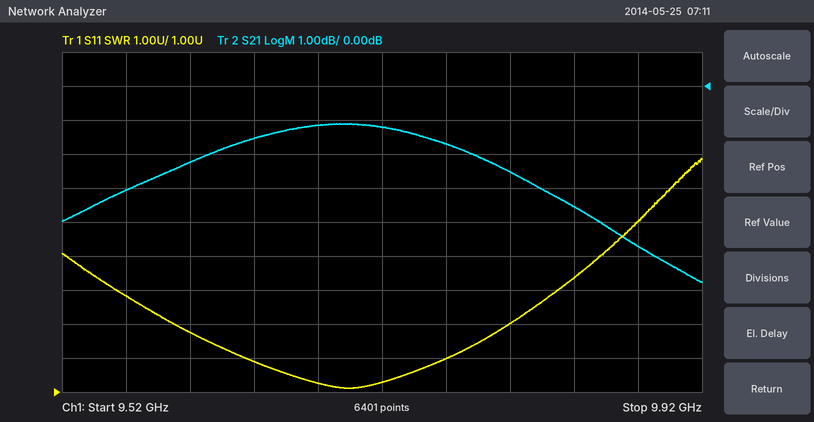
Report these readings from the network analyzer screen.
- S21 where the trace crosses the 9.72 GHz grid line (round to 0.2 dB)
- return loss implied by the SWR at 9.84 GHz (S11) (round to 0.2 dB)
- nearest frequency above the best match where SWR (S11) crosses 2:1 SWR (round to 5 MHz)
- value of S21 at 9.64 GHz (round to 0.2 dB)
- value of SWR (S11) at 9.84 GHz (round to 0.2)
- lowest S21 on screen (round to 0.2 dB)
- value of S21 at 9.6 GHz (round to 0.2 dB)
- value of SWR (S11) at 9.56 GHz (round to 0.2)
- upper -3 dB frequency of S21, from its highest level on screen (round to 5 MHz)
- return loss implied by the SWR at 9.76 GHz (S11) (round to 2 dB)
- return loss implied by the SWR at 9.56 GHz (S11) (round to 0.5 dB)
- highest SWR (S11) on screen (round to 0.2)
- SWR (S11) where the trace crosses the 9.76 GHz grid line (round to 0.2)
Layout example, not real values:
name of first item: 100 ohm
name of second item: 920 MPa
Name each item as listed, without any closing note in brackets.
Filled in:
S21 where the trace crosses the 9.72 GHz grid line: -1.2 dB
return loss implied by the SWR at 9.84 GHz (S11): 4.0 dB
nearest frequency above the best match where SWR (S11) crosses 2:1 SWR: 9.760 GHz
value of S21 at 9.64 GHz: -1.6 dB
value of SWR (S11) at 9.84 GHz: 4.4
lowest S21 on screen: -5.8 dB
value of S21 at 9.6 GHz: -2.2 dB
value of SWR (S11) at 9.56 GHz: 3.8
upper -3 dB frequency of S21, from its highest level on screen: 9.860 GHz
return loss implied by the SWR at 9.76 GHz (S11): 10 dB
return loss implied by the SWR at 9.56 GHz (S11): 4.5 dB
highest SWR (S11) on screen: 7.8
SWR (S11) where the trace crosses the 9.76 GHz grid line: 2.0
